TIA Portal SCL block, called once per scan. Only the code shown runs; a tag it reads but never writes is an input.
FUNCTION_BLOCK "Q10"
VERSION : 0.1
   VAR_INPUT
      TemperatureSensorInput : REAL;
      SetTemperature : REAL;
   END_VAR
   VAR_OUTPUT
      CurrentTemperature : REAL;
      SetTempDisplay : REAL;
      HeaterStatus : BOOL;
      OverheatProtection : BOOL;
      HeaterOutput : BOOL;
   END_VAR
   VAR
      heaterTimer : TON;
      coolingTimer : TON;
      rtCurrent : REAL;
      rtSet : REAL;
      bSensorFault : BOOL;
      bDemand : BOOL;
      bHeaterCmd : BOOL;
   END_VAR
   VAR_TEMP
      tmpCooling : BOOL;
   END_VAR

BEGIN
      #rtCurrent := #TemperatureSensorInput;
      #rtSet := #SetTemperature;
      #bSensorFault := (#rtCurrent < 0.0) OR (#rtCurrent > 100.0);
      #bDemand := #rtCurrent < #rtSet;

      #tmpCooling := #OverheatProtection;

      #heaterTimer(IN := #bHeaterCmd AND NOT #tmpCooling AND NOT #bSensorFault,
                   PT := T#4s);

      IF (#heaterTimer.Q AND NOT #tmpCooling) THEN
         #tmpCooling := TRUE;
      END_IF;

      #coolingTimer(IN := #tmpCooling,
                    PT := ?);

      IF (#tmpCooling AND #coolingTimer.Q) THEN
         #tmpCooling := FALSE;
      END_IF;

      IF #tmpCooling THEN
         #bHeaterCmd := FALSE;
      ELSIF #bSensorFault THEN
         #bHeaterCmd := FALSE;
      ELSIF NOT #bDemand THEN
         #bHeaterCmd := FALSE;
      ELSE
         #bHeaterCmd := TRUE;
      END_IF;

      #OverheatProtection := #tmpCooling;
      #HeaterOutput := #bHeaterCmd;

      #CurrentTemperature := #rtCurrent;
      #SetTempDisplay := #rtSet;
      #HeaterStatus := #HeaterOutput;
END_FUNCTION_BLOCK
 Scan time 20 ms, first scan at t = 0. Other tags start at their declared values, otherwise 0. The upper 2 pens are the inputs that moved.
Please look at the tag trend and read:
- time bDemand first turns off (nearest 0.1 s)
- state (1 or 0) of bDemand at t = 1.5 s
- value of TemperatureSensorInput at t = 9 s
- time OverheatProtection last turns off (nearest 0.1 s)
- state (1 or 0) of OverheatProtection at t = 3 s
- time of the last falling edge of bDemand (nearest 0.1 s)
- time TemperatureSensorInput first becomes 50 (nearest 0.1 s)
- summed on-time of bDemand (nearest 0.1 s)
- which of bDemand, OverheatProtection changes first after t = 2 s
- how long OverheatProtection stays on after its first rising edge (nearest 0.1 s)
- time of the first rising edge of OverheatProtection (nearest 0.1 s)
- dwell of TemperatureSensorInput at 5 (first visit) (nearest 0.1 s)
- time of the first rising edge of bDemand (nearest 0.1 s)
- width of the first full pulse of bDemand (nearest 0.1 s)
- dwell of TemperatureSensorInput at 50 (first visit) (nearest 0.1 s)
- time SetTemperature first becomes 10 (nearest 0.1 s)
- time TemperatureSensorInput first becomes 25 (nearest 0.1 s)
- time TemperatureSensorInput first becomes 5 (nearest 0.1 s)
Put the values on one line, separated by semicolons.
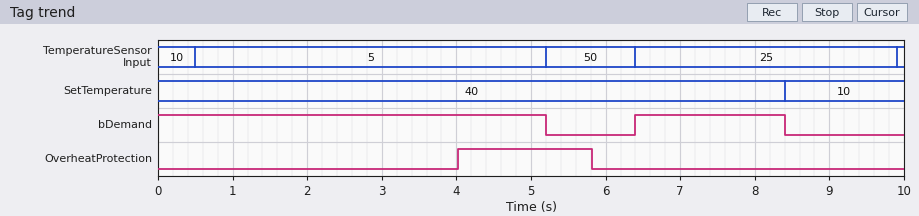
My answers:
5.2 s; 1; 25; 5.8 s; 0; 8.4 s; 5.2 s; 7.2 s; OverheatProtection; 1.8 s; 4.0 s; 4.7 s; 6.4 s; 2.0 s; 1.2 s; 8.4 s; 6.4 s; 0.5 s
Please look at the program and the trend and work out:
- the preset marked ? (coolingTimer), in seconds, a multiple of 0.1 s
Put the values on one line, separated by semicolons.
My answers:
1.8 s
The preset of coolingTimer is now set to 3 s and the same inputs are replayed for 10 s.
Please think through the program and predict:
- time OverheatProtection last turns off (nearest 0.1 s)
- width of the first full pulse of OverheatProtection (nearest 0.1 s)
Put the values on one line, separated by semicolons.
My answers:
7.0 s; 3.0 s
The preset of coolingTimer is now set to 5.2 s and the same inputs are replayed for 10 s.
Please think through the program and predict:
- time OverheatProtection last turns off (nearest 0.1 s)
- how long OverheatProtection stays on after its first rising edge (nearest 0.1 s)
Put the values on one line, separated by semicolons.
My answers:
9.2 s; 5.2 s
